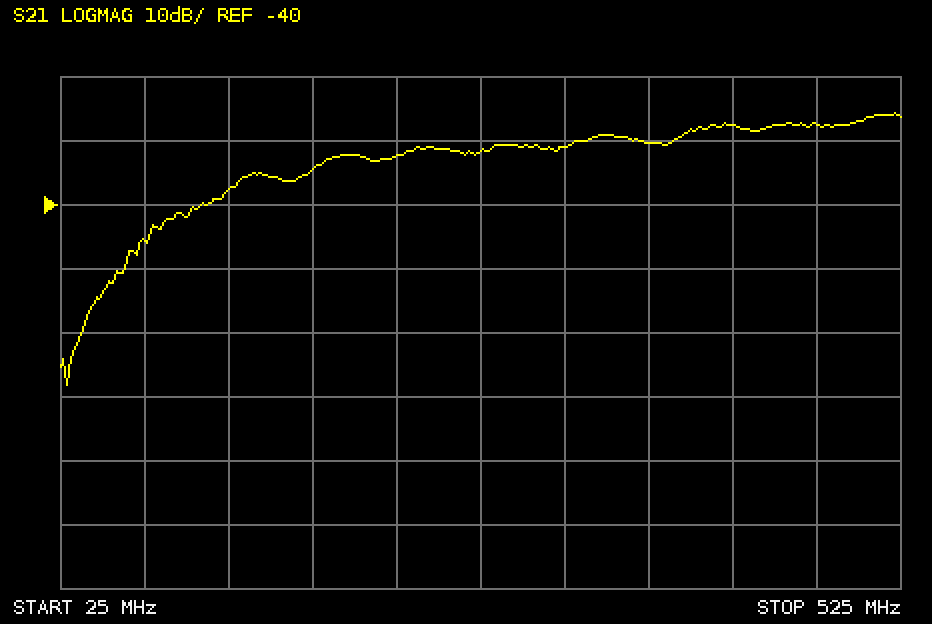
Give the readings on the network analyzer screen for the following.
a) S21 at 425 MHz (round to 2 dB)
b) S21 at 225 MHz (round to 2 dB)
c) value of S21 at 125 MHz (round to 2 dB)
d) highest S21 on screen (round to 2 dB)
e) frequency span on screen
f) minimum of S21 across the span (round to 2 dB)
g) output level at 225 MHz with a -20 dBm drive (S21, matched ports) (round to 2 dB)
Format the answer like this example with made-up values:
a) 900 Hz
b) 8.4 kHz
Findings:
a) -28 dB
b) -32 dB
c) -38 dB
d) -26 dB
e) 500 MHz
f) -68 dB
g) -52 dBm
